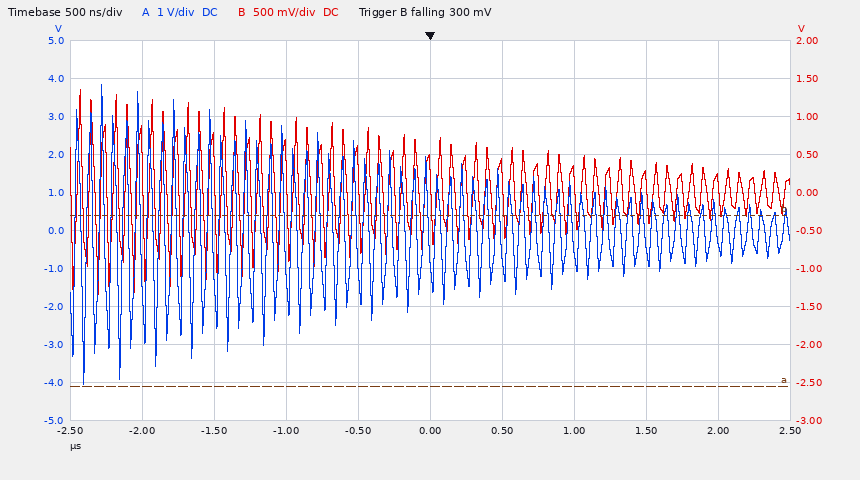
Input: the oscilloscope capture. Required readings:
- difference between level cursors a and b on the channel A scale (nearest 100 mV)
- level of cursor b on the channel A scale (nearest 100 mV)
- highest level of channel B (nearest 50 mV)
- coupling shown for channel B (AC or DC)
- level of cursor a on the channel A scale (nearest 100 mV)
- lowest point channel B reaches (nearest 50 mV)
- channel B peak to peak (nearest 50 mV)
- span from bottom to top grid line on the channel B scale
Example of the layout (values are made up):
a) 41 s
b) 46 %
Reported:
a) 4.5 V
b) 400 mV
c) 1.35 V
d) DC
e) -4.1 V
f) -1.35 V
g) 2.70 V
h) 5 V
